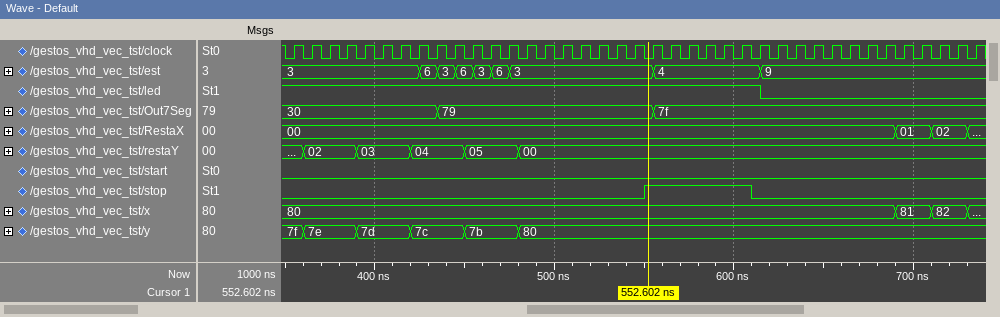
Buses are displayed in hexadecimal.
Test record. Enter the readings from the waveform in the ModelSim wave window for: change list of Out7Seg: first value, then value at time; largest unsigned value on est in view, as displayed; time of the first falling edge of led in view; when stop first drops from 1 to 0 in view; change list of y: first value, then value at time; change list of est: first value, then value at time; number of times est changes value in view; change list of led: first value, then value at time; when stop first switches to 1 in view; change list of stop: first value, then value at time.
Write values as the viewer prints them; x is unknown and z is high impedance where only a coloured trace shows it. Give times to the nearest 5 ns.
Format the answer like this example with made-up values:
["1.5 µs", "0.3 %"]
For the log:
["30, 79 at 435 ns, 7f at 555 ns", "9", "615 ns", "610 ns", "7f, 7e at 360 ns, 7d at 390 ns, 7c at 420 ns, 7b at 450 ns, 80 at 480 ns", "3, 6 at 425 ns, 3 at 435 ns, 6 at 445 ns, 3 at 455 ns, 6 at 465 ns, 3 at 475 ns, 4 at 555 ns, 9 at 615 ns", "8", "1, 0 at 615 ns", "550 ns", "0, 1 at 550 ns, 0 at 610 ns"]
